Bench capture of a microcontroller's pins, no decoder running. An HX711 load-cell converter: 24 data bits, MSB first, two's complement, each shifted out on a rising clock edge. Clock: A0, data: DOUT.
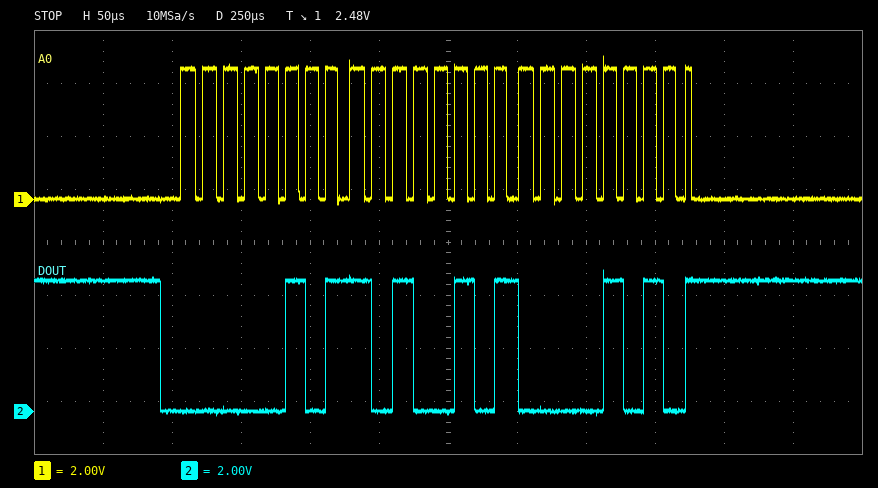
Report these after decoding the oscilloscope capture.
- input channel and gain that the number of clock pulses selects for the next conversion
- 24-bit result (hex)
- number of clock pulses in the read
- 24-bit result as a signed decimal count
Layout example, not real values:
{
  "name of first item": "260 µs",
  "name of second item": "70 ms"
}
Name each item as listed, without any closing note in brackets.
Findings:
{
  "input channel and gain that the number of clock pulses selects for the next conversion": "channel A, gain 128",
  "24-bit result": "0x05A50A",
  "number of clock pulses in the read": "25",
  "24-bit result as a signed decimal count": "369930"
}
